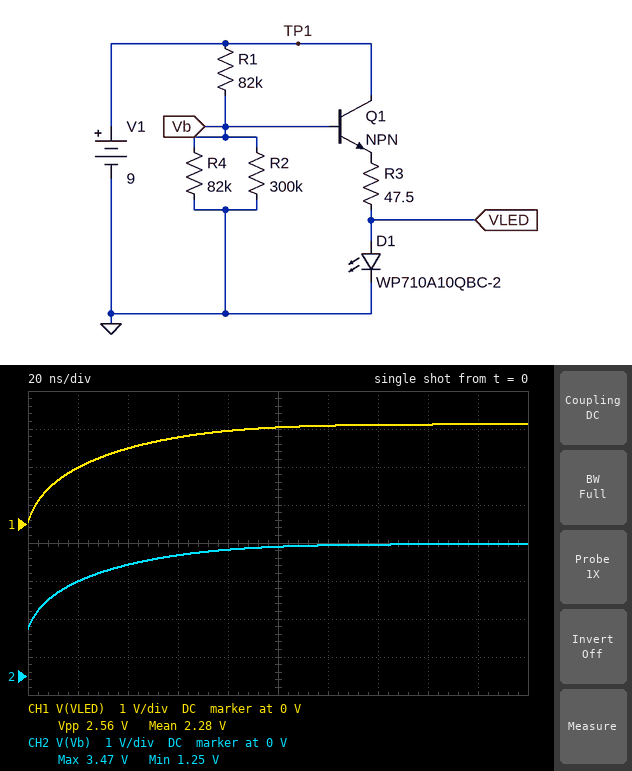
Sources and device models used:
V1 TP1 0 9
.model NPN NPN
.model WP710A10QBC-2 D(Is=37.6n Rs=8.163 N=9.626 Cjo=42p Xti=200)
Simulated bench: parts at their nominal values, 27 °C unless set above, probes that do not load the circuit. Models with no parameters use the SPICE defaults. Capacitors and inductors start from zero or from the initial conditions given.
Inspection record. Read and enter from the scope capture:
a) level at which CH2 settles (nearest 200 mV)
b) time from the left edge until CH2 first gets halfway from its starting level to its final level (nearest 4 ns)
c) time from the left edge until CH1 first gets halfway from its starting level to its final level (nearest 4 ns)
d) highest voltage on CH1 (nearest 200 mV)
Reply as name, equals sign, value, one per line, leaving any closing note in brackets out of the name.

level at which CH2 settles = 3.4 V
time from the left edge until CH2 first gets halfway from its starting level to its final level = 16 ns
time from the left edge until CH1 first gets halfway from its starting level to its final level = 16 ns
highest voltage on CH1 = 2.6 V
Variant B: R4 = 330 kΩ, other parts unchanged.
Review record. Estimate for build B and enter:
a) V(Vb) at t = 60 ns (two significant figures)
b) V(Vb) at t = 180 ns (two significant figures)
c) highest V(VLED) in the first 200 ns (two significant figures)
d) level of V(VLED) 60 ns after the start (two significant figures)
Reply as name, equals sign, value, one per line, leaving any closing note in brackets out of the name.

V(Vb) at t = 60 ns = 3.7 V
V(Vb) at t = 180 ns = 3.9 V
highest V(VLED) in the first 200 ns = 2.9 V
level of V(VLED) 60 ns after the start = 2.7 V
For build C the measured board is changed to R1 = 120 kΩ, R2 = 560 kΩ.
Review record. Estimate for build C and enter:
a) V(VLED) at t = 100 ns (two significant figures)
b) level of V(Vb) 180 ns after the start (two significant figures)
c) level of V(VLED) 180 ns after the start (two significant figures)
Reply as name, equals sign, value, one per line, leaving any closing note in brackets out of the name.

V(VLED) at t = 100 ns = 2.1 V
level of V(Vb) 180 ns after the start = 3.1 V
level of V(VLED) 180 ns after the start = 2.3 V
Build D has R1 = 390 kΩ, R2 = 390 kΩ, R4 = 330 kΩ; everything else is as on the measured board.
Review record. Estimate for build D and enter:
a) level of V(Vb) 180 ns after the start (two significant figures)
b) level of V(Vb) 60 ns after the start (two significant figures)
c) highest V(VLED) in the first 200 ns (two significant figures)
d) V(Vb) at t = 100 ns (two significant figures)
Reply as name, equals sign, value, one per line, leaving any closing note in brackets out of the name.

level of V(Vb) 180 ns after the start = 2.4 V
level of V(Vb) 60 ns after the start = 1.9 V
highest V(VLED) in the first 200 ns = 1.7 V
V(Vb) at t = 100 ns = 2.1 V
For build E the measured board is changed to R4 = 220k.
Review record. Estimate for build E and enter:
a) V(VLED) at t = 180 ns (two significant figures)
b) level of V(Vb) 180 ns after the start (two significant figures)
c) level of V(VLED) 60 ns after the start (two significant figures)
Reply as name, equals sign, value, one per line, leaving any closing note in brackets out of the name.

V(VLED) at t = 180 ns = 2.9 V
level of V(Vb) 180 ns after the start = 3.8 V
level of V(VLED) 60 ns after the start = 2.7 V
